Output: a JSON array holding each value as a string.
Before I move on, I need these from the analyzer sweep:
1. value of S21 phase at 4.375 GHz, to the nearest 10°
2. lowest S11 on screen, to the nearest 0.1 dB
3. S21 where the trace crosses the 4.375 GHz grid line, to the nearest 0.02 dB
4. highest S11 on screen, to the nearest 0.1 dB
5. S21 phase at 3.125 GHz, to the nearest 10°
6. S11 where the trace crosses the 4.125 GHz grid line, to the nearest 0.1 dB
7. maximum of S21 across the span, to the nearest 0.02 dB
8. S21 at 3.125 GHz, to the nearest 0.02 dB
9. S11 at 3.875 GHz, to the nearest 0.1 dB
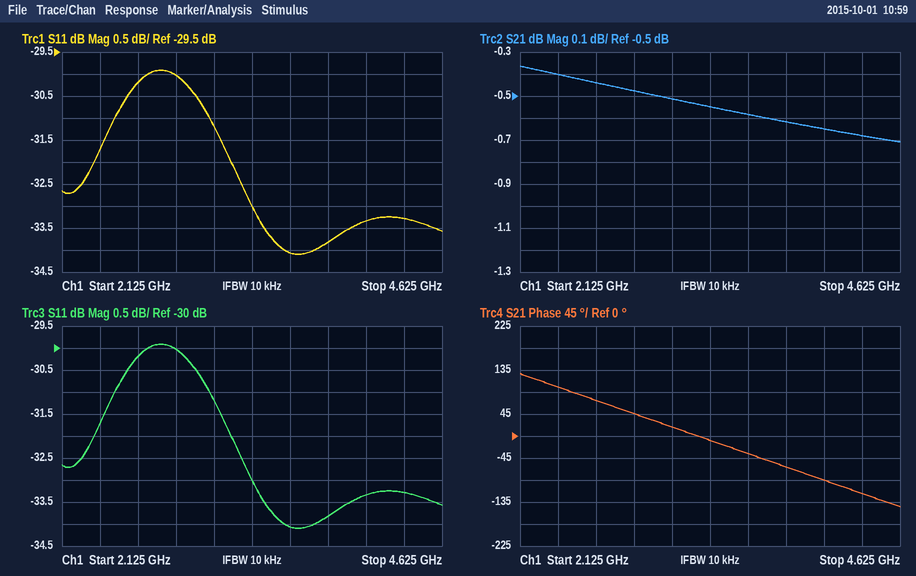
["-120°", "-34.1 dB", "-0.68 dB", "-29.9 dB", "20°", "-33.3 dB", "-0.36 dB", "-0.52 dB", "-33.8 dB"]
